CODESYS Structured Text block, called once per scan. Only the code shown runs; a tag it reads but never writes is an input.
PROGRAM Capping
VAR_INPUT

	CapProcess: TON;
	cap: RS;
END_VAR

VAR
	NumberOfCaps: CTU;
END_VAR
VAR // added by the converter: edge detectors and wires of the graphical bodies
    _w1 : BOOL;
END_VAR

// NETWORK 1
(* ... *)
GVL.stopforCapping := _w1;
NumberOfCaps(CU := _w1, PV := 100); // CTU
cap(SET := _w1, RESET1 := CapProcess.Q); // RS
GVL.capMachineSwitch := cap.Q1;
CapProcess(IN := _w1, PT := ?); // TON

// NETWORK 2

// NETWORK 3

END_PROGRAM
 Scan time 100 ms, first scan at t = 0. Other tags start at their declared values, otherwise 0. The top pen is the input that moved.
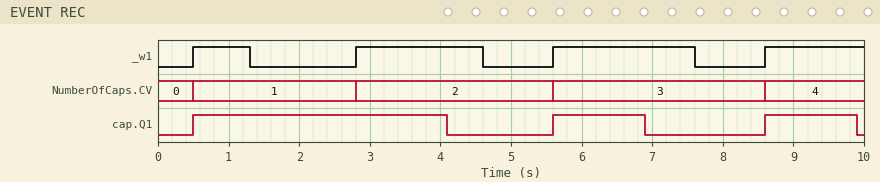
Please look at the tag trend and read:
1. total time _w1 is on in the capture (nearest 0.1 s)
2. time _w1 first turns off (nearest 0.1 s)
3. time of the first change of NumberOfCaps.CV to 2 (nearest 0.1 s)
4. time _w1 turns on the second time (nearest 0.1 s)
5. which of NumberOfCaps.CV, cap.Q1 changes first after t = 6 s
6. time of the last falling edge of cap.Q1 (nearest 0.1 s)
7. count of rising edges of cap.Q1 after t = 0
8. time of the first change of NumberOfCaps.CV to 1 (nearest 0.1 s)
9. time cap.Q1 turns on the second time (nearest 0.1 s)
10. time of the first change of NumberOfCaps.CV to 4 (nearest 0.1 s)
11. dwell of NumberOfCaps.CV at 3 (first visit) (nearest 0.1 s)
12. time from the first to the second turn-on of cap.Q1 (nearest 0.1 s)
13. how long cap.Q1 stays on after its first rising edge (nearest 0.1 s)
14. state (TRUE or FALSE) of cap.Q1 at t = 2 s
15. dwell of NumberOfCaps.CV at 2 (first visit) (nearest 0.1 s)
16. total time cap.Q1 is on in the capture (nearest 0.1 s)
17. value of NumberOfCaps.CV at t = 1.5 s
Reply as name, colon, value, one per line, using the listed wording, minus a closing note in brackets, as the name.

total time _w1 is on in the capture: 6.0 s
time _w1 first turns off: 1.3 s
time of the first change of NumberOfCaps.CV to 2: 2.8 s
time _w1 turns on the second time: 2.8 s
which of NumberOfCaps.CV, cap.Q1 changes first after t = 6 s: cap.Q1
time of the last falling edge of cap.Q1: 9.9 s
count of rising edges of cap.Q1 after t = 0: 3
time of the first change of NumberOfCaps.CV to 1: 0.5 s
time cap.Q1 turns on the second time: 5.6 s
time of the first change of NumberOfCaps.CV to 4: 8.6 s
dwell of NumberOfCaps.CV at 3 (first visit): 3.0 s
time from the first to the second turn-on of cap.Q1: 5.1 s
how long cap.Q1 stays on after its first rising edge: 3.6 s
state (TRUE or FALSE) of cap.Q1 at t = 2 s: TRUE
dwell of NumberOfCaps.CV at 2 (first visit): 2.8 s
total time cap.Q1 is on in the capture: 6.2 s
value of NumberOfCaps.CV at t = 1.5 s: 1
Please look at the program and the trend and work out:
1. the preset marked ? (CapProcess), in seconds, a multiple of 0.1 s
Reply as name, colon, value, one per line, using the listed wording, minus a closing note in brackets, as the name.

the preset marked ? (CapProcess), in seconds, a multiple of 0.1 s: 1.2 s
